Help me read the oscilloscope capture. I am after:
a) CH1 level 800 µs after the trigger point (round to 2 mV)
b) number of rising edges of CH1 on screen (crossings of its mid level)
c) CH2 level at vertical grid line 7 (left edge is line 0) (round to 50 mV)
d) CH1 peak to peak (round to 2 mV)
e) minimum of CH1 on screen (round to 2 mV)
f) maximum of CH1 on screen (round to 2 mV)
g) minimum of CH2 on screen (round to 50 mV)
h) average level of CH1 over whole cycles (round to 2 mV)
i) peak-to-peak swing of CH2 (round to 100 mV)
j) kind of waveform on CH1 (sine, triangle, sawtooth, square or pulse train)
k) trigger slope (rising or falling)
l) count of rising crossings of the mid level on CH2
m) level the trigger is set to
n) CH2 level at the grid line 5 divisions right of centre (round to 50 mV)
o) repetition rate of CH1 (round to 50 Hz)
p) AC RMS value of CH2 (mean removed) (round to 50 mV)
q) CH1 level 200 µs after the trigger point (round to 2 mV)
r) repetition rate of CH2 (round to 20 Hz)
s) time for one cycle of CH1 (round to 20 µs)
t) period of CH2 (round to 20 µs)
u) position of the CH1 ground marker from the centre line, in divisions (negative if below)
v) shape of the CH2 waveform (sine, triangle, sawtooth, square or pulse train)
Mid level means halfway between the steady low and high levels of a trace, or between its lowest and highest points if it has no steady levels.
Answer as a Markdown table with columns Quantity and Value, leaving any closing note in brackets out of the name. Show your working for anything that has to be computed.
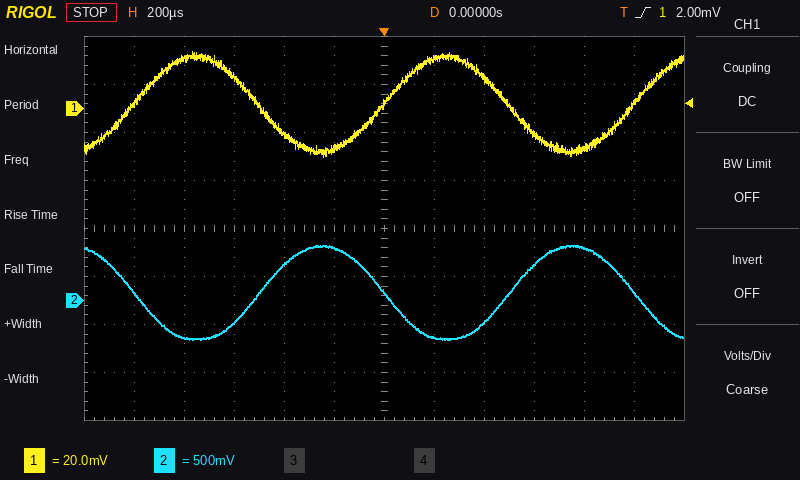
| Quantity | Value |
|---|---|
| CH1 level 800 µs after the trigger point | -16 mV |
| number of rising edges of CH1 on screen | 3 |
| CH2 level at vertical grid line 7 (left edge is line 0) | -400 mV |
| CH1 peak to peak | 24 mV − (-20 mV) = 44 mV |
| minimum of CH1 on screen | -20 mV |
| maximum of CH1 on screen | 24 mV |
| minimum of CH2 on screen | -400 mV |
| average level of CH1 over whole cycles | (24 mV + (-20 mV)) / 2 ≈ 2 mV |
| peak-to-peak swing of CH2 | 1.00 V |
| kind of waveform on CH1 | sine |
| trigger slope | rising |
| count of rising crossings of the mid level on CH2 | 2 |
| level the trigger is set to | 2.00 mV |
| CH2 level at the grid line 5 divisions right of centre | 100 mV |
| repetition rate of CH1 | 1 / 1.00 ms ≈ 1.00 kHz |
| AC RMS value of CH2 (mean removed) | 1.00 V / (2√2) ≈ 354 mV, so 350 mV to the nearest 50 mV |
| CH1 level 200 µs after the trigger point | 20 mV |
| repetition rate of CH2 | 1 / 1.00 ms ≈ 1.00 kHz |
| time for one cycle of CH1 | 1.00 ms |
| period of CH2 | 1.00 ms |
| position of the CH1 ground marker from the centre line, in divisions | +2.5 div |
| shape of the CH2 waveform | sine |
